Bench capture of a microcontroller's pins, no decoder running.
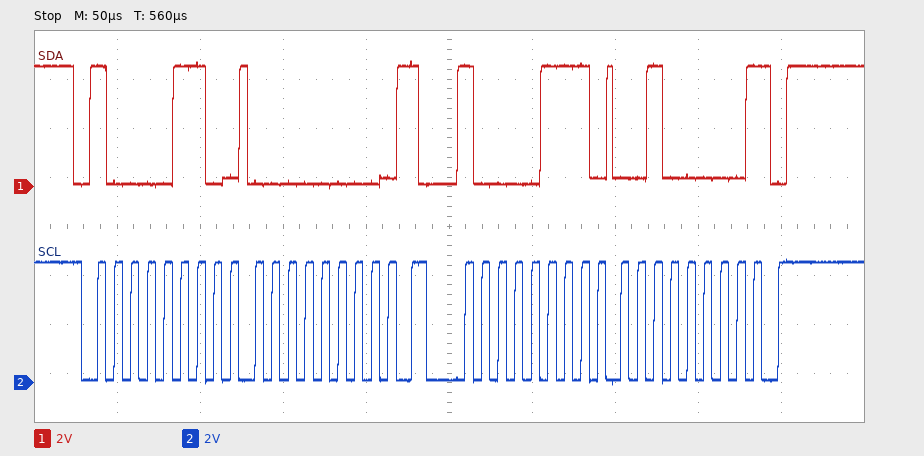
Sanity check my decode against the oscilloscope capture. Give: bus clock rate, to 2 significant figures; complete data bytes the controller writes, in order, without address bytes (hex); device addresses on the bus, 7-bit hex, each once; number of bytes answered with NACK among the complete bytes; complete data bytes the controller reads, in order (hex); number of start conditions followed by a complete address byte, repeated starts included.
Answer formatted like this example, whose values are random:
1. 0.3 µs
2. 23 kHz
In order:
1. 100 kHz
2. 00
3. 0x43
4. 1
5. 20
6. 2
